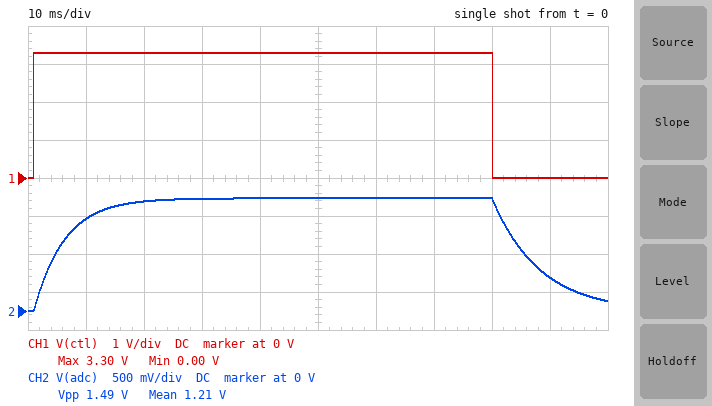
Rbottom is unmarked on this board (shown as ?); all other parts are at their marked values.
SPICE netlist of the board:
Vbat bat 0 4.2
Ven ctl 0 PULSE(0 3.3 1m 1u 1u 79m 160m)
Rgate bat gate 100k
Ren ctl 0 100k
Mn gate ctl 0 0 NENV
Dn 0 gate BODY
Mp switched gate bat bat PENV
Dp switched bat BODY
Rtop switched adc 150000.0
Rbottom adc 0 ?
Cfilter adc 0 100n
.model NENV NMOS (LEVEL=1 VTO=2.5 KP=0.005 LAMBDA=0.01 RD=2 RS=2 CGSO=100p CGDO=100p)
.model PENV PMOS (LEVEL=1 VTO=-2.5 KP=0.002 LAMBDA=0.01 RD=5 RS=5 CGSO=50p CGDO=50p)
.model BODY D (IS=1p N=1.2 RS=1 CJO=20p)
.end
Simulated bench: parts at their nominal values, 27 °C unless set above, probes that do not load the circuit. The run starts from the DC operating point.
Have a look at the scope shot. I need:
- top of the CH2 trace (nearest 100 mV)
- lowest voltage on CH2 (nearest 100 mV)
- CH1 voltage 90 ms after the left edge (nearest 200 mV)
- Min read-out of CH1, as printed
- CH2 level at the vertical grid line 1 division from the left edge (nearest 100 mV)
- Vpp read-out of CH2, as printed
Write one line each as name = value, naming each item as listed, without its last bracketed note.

top of the CH2 trace = 1.5 V
lowest voltage on CH2 = 0 V
CH1 voltage 90 ms after the left edge = 0 V
Min read-out of CH1, as printed = 0.00 V
CH2 level at the vertical grid line 1 division from the left edge = 1.2 V
Vpp read-out of CH2, as printed = 1.49 V
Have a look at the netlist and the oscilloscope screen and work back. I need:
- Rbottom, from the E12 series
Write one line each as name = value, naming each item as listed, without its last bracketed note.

Rbottom, from the E12 series = 82 kΩ
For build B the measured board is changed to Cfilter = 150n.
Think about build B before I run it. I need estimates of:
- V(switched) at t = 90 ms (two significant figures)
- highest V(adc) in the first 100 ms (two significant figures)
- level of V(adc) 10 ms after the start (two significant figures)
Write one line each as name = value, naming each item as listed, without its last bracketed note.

V(switched) at t = 90 ms = 660 mV
highest V(adc) in the first 100 ms = 1.5 V
level of V(adc) 10 ms after the start = 1.0 V
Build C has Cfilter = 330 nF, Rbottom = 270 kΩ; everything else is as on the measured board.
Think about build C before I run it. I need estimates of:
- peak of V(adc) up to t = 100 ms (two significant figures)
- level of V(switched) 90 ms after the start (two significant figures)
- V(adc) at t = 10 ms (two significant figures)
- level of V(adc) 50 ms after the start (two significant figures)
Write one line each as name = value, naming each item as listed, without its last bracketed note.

peak of V(adc) up to t = 100 ms = 2.5 V
level of V(switched) 90 ms after the start = 2.2 V
V(adc) at t = 10 ms = 660 mV
level of V(adc) 50 ms after the start = 2.1 V
